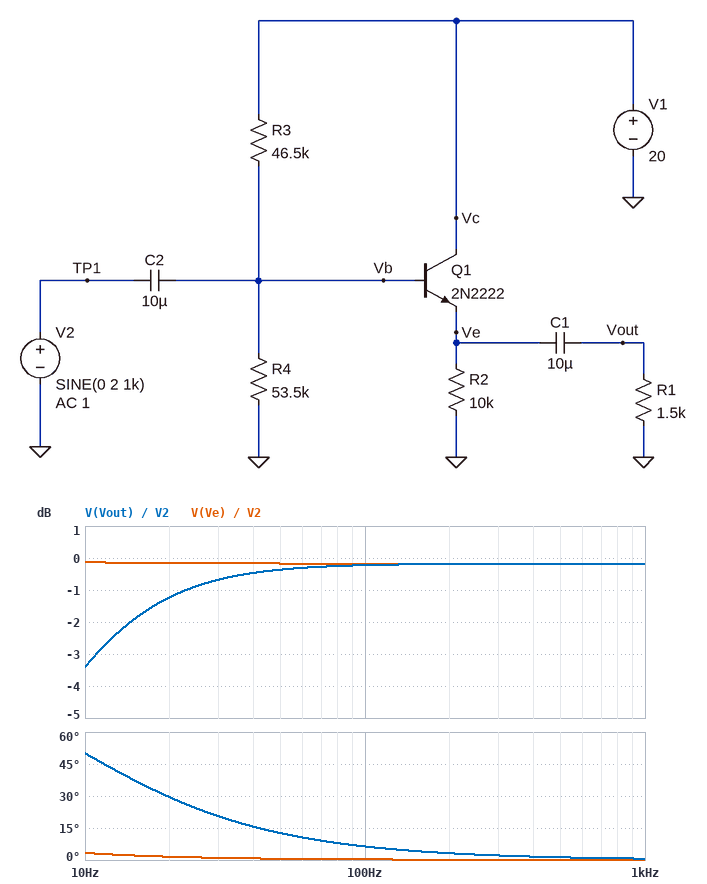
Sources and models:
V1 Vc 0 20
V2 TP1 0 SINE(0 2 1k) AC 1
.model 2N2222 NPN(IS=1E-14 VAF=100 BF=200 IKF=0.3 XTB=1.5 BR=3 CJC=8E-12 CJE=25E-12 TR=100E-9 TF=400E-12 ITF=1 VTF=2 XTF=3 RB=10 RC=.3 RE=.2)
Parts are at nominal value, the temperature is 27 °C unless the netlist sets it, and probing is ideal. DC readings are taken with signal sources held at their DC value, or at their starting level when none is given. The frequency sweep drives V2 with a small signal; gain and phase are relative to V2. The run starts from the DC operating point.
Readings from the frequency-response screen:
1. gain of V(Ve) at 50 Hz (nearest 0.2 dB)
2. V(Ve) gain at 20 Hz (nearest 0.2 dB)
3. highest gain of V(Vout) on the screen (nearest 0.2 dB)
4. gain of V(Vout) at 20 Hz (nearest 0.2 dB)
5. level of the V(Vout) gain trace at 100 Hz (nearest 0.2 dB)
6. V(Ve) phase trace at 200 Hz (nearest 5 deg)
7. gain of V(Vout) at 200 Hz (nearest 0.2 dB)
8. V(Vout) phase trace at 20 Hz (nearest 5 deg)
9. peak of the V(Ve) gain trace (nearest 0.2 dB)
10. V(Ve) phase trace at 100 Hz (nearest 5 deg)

-0.2 dB
-0.2 dB
-0.2 dB
-1.2 dB
-0.2 dB
0 deg
-0.2 dB
30 deg
-0.2 dB
0 deg
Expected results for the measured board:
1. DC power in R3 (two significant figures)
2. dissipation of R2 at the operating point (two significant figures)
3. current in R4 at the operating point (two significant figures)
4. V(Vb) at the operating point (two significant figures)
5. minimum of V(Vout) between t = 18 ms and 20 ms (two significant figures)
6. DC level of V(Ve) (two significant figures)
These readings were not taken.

1.9 mW
9.9 mW
200 µA
11 V
-1.3 V
9.9 V
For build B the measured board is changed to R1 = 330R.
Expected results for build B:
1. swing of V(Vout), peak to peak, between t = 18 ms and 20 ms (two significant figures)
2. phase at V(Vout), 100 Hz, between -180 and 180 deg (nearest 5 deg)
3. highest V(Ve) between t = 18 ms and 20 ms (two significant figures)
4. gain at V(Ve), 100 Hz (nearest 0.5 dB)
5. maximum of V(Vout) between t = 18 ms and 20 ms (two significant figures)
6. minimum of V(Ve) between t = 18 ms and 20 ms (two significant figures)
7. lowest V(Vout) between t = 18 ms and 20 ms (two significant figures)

1.4 V
25 deg
12 V
-0.5 dB
1.1 V
10 V
-350 mV
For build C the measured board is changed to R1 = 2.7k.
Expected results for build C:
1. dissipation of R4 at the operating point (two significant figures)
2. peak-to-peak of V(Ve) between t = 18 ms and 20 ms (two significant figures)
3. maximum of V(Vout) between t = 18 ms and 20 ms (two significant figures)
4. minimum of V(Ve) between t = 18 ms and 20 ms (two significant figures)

2.1 mW
3.9 V
2.0 V
8.0 V
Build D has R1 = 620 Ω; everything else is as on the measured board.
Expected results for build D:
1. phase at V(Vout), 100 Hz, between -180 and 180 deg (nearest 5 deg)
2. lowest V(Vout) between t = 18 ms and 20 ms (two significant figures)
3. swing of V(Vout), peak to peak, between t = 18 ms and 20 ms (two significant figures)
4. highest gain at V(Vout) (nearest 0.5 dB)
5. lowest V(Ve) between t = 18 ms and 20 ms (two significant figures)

15 deg
-610 mV
2.1 V
-0.5 dB
9.8 V
